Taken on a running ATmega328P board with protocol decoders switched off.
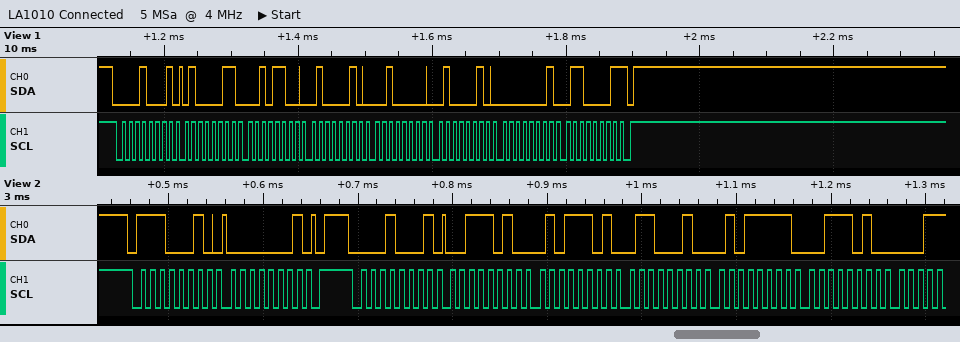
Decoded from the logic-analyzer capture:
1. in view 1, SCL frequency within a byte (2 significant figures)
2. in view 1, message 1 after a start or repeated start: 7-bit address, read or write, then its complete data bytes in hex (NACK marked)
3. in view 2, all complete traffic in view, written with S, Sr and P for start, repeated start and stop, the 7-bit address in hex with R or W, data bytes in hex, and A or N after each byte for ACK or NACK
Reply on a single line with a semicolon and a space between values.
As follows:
100 kHz; 0x08 read: 43 2C 42 20 42 01 61 NACK; S 71W A 01 A P S 08R A 3A A 5D A 62 A 5F A 3A A
